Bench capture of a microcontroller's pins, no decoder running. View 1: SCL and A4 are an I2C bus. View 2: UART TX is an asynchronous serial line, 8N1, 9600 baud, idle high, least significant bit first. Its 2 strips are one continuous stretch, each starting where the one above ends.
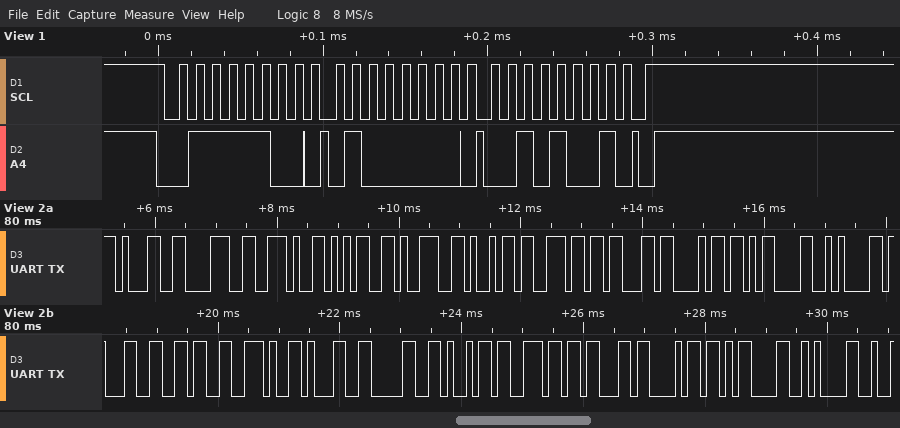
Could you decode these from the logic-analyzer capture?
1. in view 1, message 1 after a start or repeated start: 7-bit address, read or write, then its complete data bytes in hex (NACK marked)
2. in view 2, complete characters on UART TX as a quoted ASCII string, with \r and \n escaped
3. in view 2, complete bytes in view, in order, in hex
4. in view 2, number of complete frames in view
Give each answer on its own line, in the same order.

0x3E write: 40 29
"18.59inch\r\n16.10inch\r\n"
0x31 0x38 0x2E 0x35 0x39 0x69 0x6E 0x63 0x68 0x0D 0x0A 0x31 0x36 0x2E 0x31 0x30 0x69 0x6E 0x63 0x68 0x0D 0x0A
22
